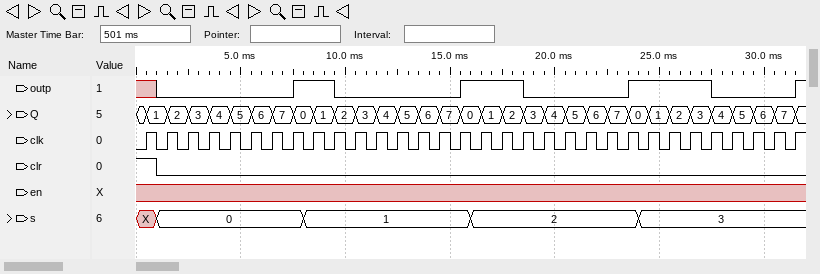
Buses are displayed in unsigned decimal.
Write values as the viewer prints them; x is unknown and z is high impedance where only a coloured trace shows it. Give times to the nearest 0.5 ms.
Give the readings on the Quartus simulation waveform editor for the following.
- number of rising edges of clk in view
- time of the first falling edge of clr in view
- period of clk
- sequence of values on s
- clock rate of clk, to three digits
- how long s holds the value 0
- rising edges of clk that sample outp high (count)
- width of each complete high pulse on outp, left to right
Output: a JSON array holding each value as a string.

["32", "1 ms", "1 ms", "X, 0, 1, 2, 3", "1.00 kHz", "7 ms", "9", "2 ms, 3 ms, 4 ms"]
